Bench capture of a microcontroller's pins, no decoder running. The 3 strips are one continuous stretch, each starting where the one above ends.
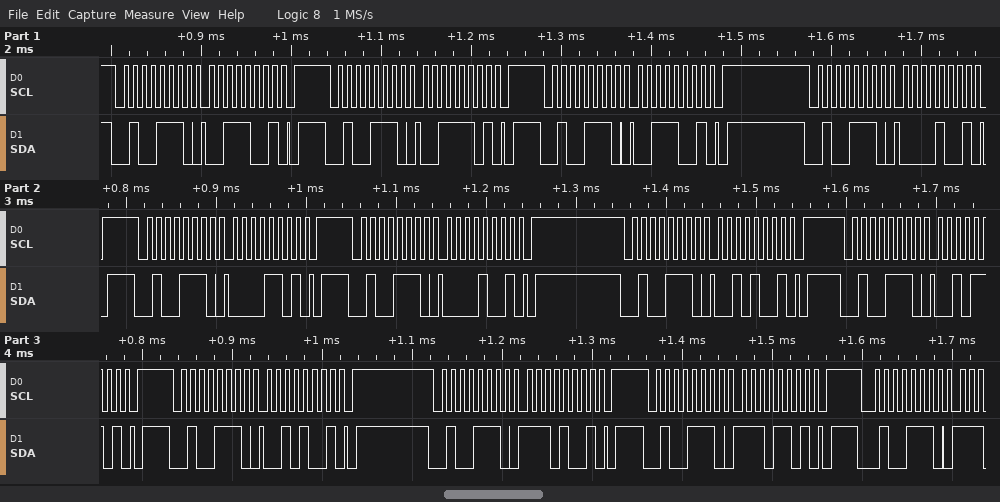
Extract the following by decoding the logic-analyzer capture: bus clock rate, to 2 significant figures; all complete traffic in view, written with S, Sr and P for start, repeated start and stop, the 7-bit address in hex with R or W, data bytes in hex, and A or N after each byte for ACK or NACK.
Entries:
100 kHz
S 27W A 39 A P S 27W A 3D A P S 27W A 39 A P S 27W A 09 A P S 27W A 0D A P S 27W A 09 A P S 27W A 29 A P S 27W A 2D A P S 27W A 29 A P S 27W A E9 A P S 27W A ED A P S 27W A
